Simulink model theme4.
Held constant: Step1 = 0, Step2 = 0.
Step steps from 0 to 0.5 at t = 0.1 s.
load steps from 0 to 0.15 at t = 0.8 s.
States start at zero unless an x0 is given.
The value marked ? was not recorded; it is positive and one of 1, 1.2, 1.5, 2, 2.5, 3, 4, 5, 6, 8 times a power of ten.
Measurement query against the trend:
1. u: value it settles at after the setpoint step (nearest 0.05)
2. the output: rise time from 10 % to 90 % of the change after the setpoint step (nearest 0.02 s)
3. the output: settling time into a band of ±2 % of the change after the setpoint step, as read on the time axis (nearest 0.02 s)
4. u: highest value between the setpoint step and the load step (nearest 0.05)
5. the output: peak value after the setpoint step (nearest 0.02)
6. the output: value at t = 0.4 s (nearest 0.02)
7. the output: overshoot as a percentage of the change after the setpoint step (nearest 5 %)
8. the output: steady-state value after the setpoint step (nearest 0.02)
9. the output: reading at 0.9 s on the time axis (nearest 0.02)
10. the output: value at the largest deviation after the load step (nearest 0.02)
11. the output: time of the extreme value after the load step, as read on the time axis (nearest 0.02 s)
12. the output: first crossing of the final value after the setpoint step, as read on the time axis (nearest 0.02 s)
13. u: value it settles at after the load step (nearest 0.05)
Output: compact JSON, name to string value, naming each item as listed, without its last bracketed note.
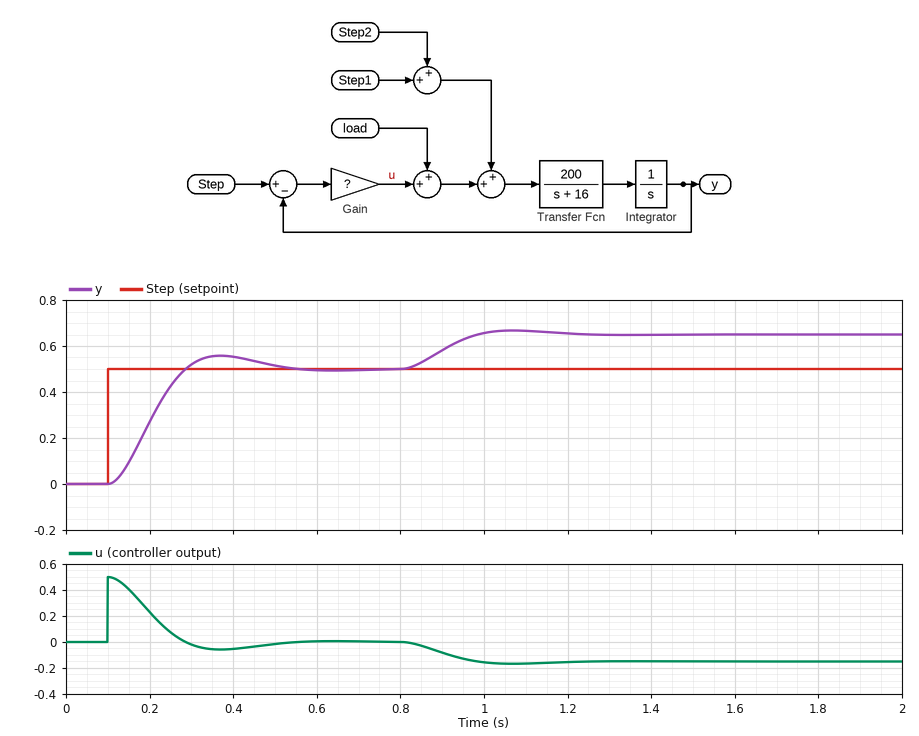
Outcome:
{"u: value it settles at after the setpoint step": "0.00", "the output: rise time from 10 % to 90 % of the change after the setpoint step": "0.12 s", "the output: settling time into a band of ±2 % of the change after the setpoint step, as read on the time axis": "0.52 s", "u: highest value between the setpoint step and the load step": "0.50", "the output: peak value after the setpoint step": "0.56", "the output: value at t = 0.4 s": "0.56", "the output: overshoot as a percentage of the change after the setpoint step": "10 %", "the output: steady-state value after the setpoint step": "0.50", "the output: reading at 0.9 s on the time axis": "0.58", "the output: value at the largest deviation after the load step": "0.66", "the output: time of the extreme value after the load step, as read on the time axis": "1.06 s", "the output: first crossing of the final value after the setpoint step, as read on the time axis": "0.28 s", "u: value it settles at after the load step": "-0.15"}
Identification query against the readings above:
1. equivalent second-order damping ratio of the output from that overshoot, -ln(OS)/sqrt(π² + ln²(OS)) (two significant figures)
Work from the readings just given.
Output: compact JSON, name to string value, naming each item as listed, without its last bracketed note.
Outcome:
{"equivalent second-order damping ratio of the output from that overshoot, -ln(OS)/sqrt(π² + ln²(OS))": "0.59"}
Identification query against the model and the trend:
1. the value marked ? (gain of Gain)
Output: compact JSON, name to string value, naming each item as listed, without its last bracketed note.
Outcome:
{"the value marked ?": "1"}
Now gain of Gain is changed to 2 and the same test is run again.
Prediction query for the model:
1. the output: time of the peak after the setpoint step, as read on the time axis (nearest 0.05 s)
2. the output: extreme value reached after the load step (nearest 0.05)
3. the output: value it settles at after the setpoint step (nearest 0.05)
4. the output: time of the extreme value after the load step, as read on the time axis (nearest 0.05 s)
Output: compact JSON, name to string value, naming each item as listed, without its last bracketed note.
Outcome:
{"the output: time of the peak after the setpoint step, as read on the time axis": "0.25 s", "the output: extreme value reached after the load step": "0.60", "the output: value it settles at after the setpoint step": "0.50", "the output: time of the extreme value after the load step, as read on the time axis": "0.95 s"}
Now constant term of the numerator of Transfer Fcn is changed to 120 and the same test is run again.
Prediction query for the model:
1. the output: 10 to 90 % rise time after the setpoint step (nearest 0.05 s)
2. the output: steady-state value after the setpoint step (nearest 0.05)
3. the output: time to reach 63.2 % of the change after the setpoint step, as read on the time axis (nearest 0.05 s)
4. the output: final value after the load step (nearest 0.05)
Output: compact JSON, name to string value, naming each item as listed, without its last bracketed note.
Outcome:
{"the output: 10 to 90 % rise time after the setpoint step": "0.20 s", "the output: steady-state value after the setpoint step": "0.50", "the output: time to reach 63.2 % of the change after the setpoint step, as read on the time axis": "0.25 s", "the output: final value after the load step": "0.65"}
